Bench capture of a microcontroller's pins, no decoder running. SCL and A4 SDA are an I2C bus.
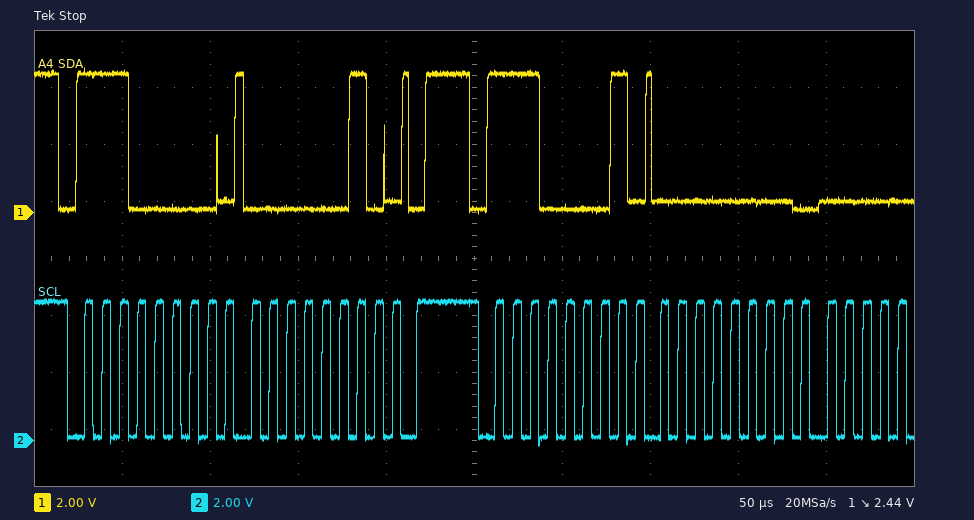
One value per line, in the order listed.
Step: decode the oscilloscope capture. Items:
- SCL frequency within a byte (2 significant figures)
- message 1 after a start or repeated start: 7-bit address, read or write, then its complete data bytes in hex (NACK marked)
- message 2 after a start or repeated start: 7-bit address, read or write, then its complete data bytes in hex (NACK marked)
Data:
100 kHz
0x70 write: 02
0x70 read: 00
